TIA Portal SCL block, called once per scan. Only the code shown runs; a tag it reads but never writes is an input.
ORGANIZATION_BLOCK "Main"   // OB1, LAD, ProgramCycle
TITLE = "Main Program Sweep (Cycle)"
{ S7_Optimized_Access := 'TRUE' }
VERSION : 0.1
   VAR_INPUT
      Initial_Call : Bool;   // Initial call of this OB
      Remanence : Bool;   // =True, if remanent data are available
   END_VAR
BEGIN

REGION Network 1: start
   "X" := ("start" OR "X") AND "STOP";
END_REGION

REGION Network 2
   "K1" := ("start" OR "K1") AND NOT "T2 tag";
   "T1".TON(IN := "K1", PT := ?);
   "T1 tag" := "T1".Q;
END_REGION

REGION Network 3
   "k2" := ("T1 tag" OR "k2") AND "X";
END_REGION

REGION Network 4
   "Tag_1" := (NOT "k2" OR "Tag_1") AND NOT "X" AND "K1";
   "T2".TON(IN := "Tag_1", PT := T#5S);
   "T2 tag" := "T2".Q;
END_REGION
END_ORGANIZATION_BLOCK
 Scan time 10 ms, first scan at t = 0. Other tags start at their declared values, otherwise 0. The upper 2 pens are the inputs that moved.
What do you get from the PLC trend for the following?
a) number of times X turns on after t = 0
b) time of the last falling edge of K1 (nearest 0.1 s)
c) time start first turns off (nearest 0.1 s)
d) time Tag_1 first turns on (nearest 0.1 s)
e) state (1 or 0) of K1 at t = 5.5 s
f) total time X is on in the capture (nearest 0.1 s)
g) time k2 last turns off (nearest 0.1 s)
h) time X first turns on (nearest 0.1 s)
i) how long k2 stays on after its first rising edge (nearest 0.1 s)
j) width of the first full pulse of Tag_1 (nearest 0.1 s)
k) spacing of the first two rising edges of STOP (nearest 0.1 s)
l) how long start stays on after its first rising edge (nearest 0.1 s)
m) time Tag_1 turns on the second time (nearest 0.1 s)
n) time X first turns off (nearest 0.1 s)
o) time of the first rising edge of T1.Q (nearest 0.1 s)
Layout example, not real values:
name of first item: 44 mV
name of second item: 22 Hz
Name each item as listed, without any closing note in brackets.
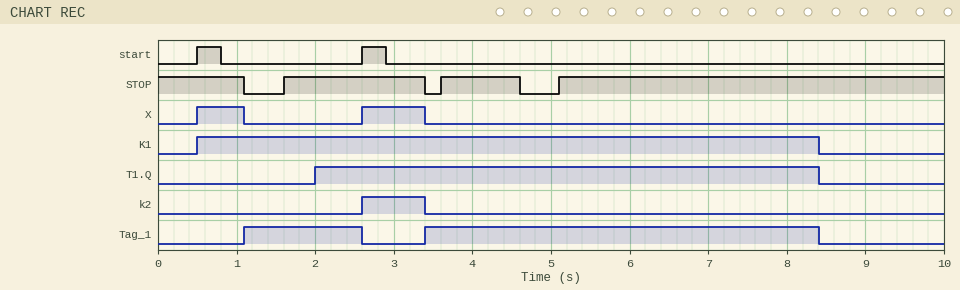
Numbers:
number of times X turns on after t = 0: 2
time of the last falling edge of K1: 8.4 s
time start first turns off: 0.8 s
time Tag_1 first turns on: 1.1 s
state (1 or 0) of K1 at t = 5.5 s: 1
total time X is on in the capture: 1.4 s
time k2 last turns off: 3.4 s
time X first turns on: 0.5 s
how long k2 stays on after its first rising edge: 0.8 s
width of the first full pulse of Tag_1: 1.5 s
spacing of the first two rising edges of STOP: 2.0 s
how long start stays on after its first rising edge: 0.3 s
time Tag_1 turns on the second time: 3.4 s
time X first turns off: 1.1 s
time of the first rising edge of T1.Q: 2.0 s
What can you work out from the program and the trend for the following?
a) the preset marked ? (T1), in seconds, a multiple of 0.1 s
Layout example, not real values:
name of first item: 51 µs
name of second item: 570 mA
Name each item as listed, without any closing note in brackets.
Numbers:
the preset marked ? (T1), in seconds, a multiple of 0.1 s: 1.5 s
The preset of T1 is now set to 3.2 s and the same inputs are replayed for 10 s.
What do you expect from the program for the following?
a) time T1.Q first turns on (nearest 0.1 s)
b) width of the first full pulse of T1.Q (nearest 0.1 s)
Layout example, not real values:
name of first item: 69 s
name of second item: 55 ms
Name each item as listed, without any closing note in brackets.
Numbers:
time T1.Q first turns on: 3.7 s
width of the first full pulse of T1.Q: 4.7 s
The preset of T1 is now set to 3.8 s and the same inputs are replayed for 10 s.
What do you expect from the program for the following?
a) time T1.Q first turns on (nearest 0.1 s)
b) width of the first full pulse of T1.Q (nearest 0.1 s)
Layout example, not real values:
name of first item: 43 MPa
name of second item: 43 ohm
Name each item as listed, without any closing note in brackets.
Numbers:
time T1.Q first turns on: 4.3 s
width of the first full pulse of T1.Q: 4.1 s
